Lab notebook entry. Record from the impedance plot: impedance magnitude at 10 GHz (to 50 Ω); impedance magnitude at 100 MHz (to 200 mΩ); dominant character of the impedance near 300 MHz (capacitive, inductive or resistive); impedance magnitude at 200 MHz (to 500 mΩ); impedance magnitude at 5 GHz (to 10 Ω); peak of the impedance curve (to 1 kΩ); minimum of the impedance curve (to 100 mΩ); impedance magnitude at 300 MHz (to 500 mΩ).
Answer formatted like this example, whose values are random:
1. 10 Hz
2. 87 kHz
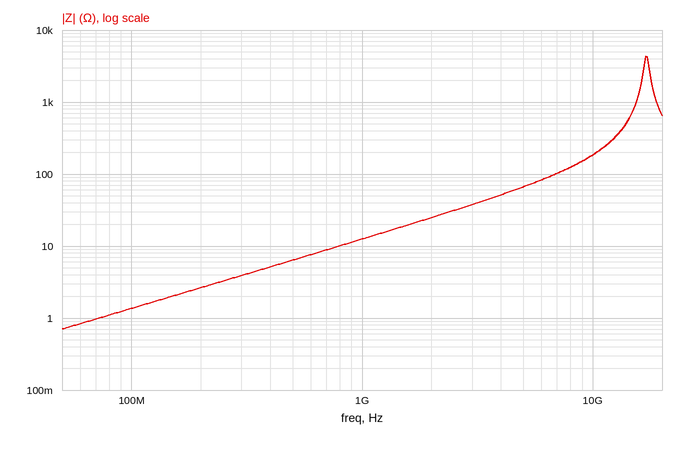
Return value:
1. 200 Ω
2. 1.4 Ω
3. inductive
4. 2.5 Ω
5. 70 Ω
6. 4 kΩ
7. 700 mΩ
8. 4.0 Ω
